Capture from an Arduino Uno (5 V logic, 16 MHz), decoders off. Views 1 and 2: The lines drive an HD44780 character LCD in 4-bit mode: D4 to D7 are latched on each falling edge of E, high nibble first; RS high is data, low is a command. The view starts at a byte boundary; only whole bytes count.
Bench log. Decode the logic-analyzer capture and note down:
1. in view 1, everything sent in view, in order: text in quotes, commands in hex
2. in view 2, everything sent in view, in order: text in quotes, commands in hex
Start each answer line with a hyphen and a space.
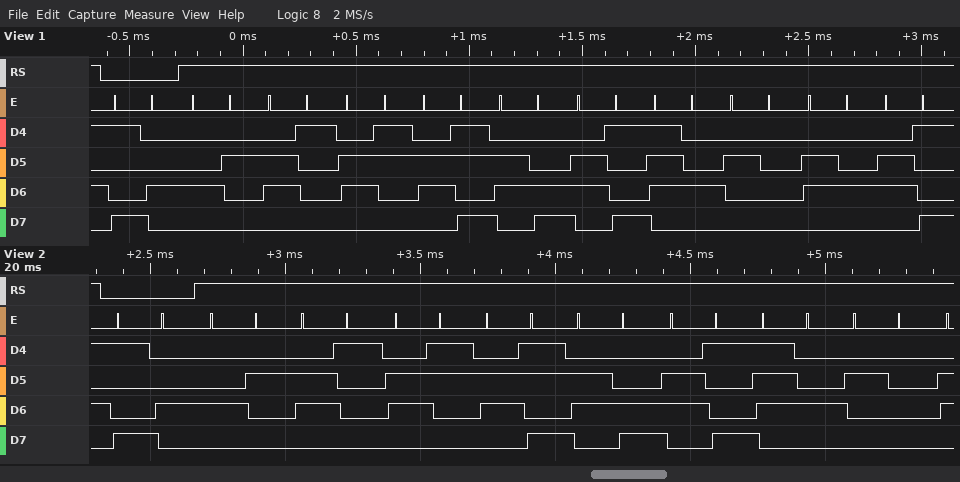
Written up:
- 0x94 "Backlit di"
- 0x94 "Backlit "
